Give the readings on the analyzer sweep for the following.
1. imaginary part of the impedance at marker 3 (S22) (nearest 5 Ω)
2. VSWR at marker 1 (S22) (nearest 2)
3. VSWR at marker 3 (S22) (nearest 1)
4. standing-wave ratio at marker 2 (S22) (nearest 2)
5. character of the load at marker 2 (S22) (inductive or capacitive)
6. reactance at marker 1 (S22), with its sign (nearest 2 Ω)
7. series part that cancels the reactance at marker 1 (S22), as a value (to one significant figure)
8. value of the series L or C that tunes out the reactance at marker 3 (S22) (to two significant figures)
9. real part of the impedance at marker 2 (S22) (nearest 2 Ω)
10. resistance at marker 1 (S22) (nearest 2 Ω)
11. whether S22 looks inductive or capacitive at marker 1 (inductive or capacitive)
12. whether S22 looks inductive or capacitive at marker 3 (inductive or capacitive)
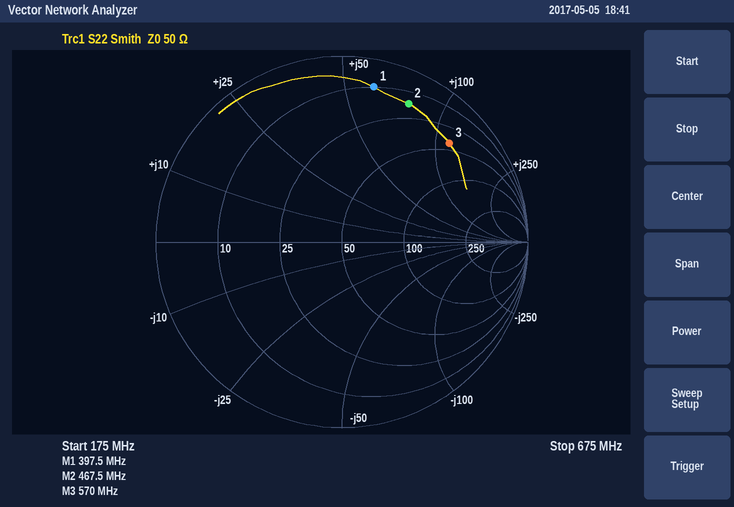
+115 Ω
12
8
10
inductive
+60 Ω
7 pF
2.4 pF
16 Ω
10 Ω
inductive
inductive
